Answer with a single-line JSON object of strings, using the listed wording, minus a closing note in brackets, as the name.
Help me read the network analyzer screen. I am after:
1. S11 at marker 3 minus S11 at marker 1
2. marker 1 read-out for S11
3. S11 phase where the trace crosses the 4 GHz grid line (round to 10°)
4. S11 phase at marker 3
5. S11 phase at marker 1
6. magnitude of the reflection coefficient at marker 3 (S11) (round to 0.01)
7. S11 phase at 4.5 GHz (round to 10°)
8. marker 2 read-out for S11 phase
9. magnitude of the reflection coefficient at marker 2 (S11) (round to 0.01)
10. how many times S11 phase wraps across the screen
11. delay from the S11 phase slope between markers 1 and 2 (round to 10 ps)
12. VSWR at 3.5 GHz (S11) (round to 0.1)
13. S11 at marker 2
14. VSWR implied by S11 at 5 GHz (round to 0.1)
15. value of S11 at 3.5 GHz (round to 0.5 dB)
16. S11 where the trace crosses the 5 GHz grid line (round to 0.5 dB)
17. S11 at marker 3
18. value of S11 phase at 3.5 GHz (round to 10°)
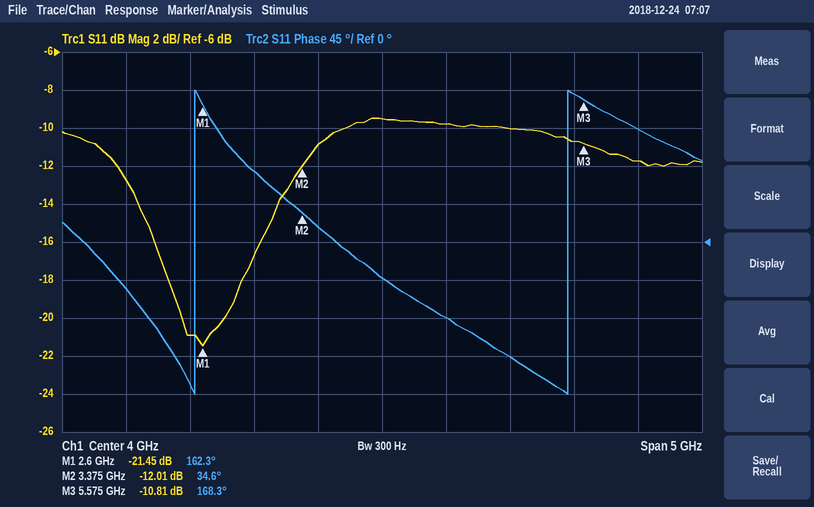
{"S11 at marker 3 minus S11 at marker 1": "10.64 dB", "marker 1 read-out for S11": "-21.45 dB", "S11 phase where the trace crosses the 4 GHz grid line": "-40°", "S11 phase at marker 3": "168.3°", "S11 phase at marker 1": "162.3°", "magnitude of the reflection coefficient at marker 3 (S11)": "0.29", "S11 phase at 4.5 GHz": "-90°", "marker 2 read-out for S11 phase": "34.6°", "magnitude of the reflection coefficient at marker 2 (S11)": "0.25", "how many times S11 phase wraps across the screen": "2", "delay from the S11 phase slope between markers 1 and 2": "460 ps", "VSWR at 3.5 GHz (S11)": "1.8", "S11 at marker 2": "-12.01 dB", "VSWR implied by S11 at 5 GHz": "1.9", "value of S11 at 3.5 GHz": "-11.0 dB", "S11 where the trace crosses the 5 GHz grid line": "-10.0 dB", "S11 at marker 3": "-10.81 dB", "value of S11 phase at 3.5 GHz": "20°"}
